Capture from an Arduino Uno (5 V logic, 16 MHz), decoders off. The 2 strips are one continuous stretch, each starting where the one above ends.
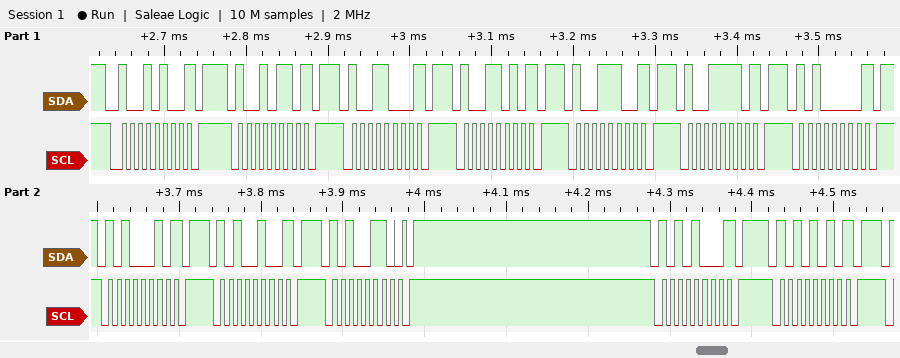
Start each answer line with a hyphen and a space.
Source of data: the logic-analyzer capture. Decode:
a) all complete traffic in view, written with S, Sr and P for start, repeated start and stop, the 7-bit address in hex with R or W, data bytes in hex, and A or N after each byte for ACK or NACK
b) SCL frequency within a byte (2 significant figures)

- S 4AW N P S 4BW N P S 4CW N P S 4DW N P S 4EW N P S 4FW N P S 50W N P S 51W N P S 52W N P S 53W A P S 54W N P S 55W N P
- 100 kHz
